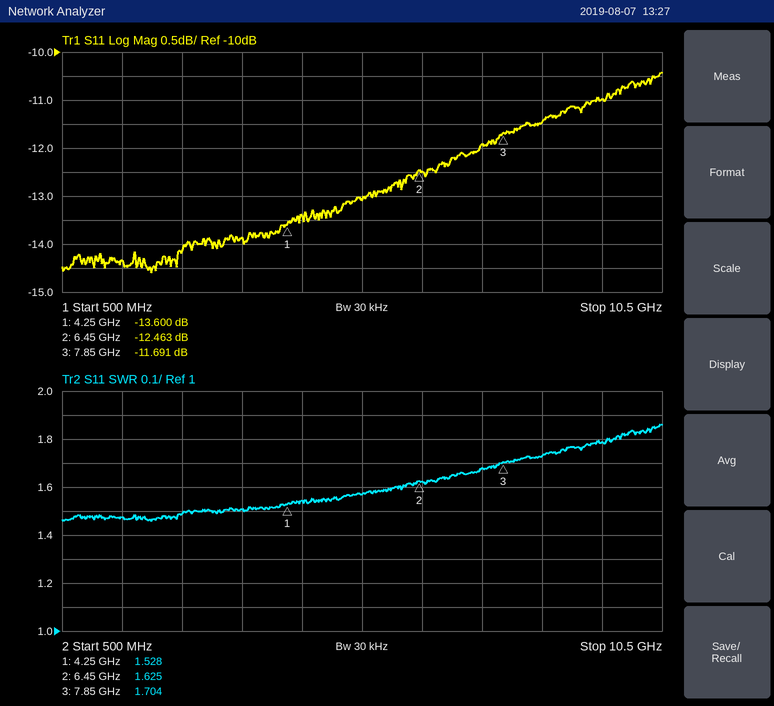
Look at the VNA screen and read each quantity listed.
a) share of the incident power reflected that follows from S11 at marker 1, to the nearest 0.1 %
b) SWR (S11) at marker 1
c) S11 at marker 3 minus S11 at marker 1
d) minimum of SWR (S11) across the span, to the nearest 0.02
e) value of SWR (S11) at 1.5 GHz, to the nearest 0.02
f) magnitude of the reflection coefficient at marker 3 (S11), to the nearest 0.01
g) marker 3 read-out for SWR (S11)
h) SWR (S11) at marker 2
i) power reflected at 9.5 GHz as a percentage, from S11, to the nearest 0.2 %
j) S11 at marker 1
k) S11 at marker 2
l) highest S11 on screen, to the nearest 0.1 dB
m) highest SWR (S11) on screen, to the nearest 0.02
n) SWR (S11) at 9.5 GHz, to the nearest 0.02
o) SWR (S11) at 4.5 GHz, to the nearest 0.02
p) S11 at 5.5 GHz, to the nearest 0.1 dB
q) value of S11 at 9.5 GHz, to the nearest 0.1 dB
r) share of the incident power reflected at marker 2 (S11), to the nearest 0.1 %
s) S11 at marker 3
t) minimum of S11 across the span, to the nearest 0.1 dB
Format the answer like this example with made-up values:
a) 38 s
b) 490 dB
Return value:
a) 4.4 %
b) 1.528
c) 1.909 dB
d) 1.46
e) 1.48
f) 0.26
g) 1.704
h) 1.625
i) 8.0 %
j) -13.600 dB
k) -12.463 dB
l) -10.4 dB
m) 1.86
n) 1.78
o) 1.54
p) -13.1 dB
q) -11.0 dB
r) 5.7 %
s) -11.691 dB
t) -14.6 dB
